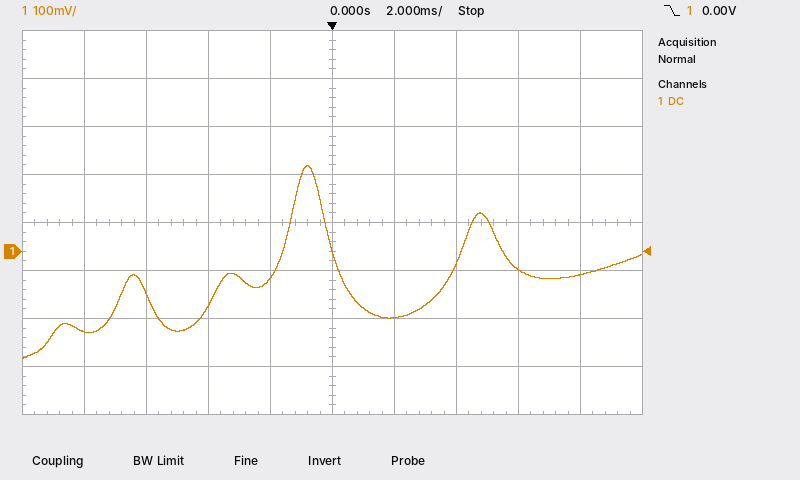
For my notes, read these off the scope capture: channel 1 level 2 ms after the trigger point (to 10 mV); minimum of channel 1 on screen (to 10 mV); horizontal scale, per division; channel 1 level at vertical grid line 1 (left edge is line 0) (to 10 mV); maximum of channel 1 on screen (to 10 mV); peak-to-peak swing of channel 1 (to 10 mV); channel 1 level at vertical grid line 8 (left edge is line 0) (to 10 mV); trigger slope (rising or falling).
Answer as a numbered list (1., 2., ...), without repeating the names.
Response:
1. -140 mV
2. -220 mV
3. 2 ms
4. -170 mV
5. 180 mV
6. 400 mV
7. -40 mV
8. falling
